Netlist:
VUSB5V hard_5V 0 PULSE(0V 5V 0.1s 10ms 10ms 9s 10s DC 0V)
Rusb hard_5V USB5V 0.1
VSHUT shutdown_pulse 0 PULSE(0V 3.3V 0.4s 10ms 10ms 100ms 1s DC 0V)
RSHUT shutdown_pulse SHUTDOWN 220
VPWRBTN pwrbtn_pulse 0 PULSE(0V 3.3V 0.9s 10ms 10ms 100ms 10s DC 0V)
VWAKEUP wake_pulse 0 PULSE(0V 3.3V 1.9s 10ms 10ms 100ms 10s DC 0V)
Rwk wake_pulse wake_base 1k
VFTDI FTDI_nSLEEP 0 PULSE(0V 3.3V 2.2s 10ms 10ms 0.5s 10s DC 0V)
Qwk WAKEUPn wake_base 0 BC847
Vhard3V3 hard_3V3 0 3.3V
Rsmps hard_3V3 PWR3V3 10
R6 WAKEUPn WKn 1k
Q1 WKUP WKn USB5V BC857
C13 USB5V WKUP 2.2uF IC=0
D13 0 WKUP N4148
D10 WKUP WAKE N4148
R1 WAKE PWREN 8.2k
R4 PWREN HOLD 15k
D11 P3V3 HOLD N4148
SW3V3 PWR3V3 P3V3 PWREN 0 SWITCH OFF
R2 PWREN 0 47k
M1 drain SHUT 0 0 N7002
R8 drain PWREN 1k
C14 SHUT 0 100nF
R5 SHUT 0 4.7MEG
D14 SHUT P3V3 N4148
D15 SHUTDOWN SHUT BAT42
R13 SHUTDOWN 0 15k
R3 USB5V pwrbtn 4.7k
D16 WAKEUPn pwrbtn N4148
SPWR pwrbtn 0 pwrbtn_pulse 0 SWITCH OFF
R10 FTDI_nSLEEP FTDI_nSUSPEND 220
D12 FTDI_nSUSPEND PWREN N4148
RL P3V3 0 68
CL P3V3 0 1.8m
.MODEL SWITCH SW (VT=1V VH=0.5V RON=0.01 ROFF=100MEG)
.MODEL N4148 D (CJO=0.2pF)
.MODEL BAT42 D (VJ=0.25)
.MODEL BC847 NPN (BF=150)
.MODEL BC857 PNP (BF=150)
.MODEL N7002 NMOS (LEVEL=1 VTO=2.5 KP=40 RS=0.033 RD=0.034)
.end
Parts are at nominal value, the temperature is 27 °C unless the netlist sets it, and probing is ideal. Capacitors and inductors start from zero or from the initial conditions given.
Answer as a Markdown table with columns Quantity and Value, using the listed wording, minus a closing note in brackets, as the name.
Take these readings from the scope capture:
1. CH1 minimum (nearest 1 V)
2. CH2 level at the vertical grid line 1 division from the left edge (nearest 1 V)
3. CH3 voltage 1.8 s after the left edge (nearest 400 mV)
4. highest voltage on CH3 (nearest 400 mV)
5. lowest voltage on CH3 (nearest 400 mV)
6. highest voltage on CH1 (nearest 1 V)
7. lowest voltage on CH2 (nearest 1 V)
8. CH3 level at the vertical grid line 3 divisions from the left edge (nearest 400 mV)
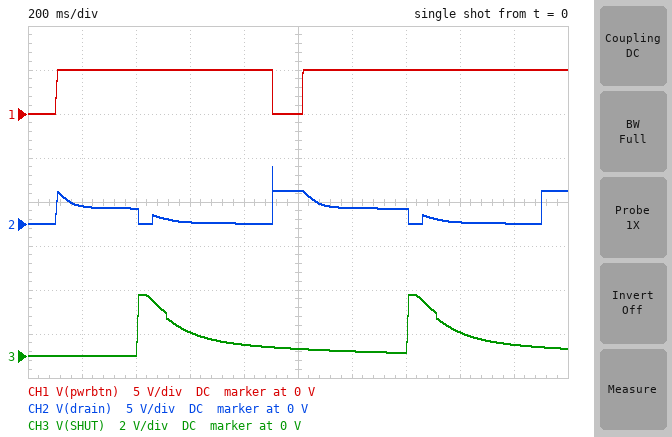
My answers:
| Quantity | Value |
|---|---|
| CH1 minimum | 0 V |
| CH2 level at the vertical grid line 1 division from the left edge | 2 V |
| CH3 voltage 1.8 s after the left edge | 400 mV |
| highest voltage on CH3 | 2.8 V |
| lowest voltage on CH3 | 0 V |
| highest voltage on CH1 | 5 V |
| lowest voltage on CH2 | 0 V |
| CH3 level at the vertical grid line 3 divisions from the left edge | 1.2 V |
